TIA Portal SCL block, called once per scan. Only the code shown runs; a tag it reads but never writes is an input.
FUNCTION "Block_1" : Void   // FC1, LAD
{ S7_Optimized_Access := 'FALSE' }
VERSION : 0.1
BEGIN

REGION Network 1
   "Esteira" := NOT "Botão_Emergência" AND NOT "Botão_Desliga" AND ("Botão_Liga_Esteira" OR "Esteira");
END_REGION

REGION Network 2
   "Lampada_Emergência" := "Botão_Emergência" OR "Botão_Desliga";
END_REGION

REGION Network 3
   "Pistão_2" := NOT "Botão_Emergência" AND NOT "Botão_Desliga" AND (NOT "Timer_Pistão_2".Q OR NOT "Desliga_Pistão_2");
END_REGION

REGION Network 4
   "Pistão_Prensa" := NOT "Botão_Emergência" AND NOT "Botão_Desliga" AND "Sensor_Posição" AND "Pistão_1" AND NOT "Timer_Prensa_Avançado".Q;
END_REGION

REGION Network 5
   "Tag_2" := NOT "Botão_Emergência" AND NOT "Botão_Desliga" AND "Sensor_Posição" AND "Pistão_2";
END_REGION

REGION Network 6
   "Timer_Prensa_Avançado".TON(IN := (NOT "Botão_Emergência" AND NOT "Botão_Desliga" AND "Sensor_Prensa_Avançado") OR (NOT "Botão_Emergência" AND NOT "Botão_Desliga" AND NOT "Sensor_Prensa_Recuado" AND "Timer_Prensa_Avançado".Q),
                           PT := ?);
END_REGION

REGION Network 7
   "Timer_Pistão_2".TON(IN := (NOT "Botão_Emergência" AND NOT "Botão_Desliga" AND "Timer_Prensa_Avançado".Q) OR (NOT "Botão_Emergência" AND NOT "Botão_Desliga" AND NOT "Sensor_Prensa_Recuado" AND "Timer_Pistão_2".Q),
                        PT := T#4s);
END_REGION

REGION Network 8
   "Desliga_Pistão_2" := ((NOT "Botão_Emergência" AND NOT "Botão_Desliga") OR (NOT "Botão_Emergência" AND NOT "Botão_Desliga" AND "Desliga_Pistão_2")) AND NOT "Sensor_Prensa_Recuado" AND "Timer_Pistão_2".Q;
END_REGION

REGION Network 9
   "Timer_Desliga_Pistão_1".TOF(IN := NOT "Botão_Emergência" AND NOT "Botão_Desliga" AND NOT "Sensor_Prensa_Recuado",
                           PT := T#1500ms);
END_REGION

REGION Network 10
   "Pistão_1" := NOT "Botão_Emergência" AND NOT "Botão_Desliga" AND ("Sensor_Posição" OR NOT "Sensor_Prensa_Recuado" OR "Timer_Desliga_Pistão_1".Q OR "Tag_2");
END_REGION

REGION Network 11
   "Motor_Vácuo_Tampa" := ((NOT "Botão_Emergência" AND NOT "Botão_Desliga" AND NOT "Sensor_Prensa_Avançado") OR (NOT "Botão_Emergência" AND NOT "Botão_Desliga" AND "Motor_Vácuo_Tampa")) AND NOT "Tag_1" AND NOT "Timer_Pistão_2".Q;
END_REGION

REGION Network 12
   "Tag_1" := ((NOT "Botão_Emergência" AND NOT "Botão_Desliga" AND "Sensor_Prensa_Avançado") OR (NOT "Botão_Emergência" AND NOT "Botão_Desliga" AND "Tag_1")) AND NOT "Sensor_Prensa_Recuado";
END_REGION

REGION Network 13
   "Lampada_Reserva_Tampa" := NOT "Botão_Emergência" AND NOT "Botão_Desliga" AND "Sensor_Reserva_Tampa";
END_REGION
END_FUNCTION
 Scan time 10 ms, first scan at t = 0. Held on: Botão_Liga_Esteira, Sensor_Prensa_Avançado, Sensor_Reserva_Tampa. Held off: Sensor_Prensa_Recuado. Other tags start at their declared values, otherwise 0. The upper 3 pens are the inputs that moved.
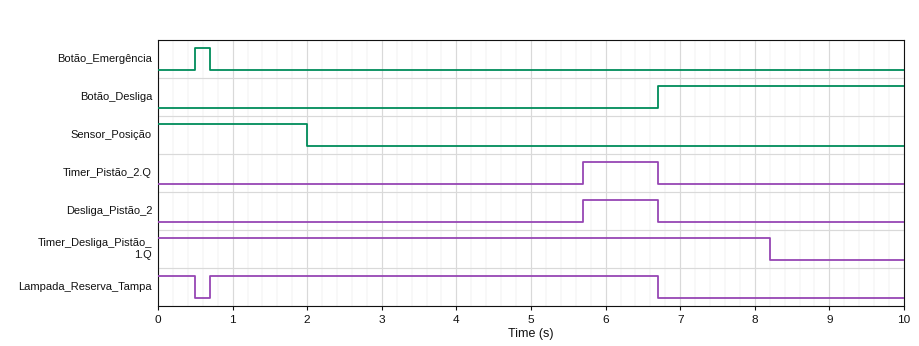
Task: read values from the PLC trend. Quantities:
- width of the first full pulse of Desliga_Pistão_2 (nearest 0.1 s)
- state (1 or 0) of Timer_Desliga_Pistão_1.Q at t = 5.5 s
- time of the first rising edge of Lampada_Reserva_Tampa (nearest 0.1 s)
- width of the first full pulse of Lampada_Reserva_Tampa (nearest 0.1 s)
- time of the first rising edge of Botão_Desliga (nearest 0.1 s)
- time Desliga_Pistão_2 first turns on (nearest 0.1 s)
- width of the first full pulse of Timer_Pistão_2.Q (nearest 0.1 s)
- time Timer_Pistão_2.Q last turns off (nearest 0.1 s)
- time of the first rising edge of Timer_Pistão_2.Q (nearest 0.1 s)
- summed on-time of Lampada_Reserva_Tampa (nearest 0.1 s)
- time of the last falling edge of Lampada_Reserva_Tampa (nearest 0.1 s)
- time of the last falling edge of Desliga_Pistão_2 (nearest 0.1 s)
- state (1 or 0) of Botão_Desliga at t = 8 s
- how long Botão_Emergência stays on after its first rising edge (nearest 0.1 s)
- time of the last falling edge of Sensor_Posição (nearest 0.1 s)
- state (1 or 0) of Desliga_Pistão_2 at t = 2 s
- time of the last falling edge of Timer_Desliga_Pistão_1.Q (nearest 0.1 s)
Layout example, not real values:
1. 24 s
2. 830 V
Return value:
1. 1.0 s
2. 1
3. 0.7 s
4. 6.0 s
5. 6.7 s
6. 5.7 s
7. 1.0 s
8. 6.7 s
9. 5.7 s
10. 6.5 s
11. 6.7 s
12. 6.7 s
13. 1
14. 0.2 s
15. 2.0 s
16. 0
17. 8.2 s
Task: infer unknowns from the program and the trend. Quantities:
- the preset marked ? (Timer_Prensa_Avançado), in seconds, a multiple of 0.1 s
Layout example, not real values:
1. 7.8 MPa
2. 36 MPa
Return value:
1. 1.0 s
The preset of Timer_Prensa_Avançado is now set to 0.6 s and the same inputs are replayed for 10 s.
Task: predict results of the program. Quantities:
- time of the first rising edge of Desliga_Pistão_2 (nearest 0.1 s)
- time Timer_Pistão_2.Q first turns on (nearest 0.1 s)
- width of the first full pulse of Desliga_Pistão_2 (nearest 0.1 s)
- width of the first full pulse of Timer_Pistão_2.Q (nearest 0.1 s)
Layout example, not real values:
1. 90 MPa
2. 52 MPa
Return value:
1. 5.3 s
2. 5.3 s
3. 1.4 s
4. 1.4 s
